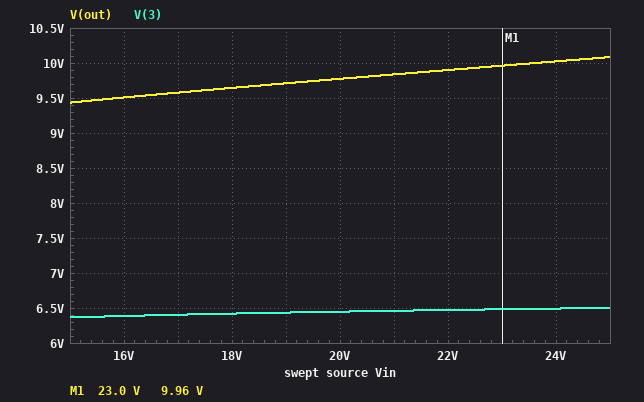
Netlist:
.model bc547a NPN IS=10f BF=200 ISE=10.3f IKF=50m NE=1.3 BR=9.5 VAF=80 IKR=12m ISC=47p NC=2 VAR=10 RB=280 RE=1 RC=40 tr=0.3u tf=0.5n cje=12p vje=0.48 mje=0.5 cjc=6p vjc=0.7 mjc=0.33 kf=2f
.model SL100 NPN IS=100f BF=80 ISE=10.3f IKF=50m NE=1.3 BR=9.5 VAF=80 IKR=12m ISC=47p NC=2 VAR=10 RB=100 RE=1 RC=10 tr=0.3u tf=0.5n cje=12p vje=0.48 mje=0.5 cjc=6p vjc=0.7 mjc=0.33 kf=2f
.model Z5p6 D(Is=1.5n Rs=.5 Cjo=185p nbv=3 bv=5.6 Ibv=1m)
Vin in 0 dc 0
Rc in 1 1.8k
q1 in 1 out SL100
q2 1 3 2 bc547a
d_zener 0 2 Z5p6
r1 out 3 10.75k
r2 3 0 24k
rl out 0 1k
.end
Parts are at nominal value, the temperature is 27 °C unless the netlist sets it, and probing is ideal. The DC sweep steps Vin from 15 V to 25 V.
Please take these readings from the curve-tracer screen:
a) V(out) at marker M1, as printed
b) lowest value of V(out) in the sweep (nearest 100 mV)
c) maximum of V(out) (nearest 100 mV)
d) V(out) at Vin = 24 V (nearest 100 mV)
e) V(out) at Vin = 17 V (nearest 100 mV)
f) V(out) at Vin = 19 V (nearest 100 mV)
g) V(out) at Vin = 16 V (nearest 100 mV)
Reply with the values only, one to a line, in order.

9.96 V
9.4 V
10.1 V
10.0 V
9.6 V
9.7 V
9.5 V
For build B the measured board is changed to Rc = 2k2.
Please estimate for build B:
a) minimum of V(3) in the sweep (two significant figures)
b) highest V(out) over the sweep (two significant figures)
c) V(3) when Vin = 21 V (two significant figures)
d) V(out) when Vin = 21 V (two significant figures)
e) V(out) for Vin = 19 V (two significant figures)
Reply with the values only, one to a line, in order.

6.3 V
9.9 V
6.4 V
9.7 V
9.6 V
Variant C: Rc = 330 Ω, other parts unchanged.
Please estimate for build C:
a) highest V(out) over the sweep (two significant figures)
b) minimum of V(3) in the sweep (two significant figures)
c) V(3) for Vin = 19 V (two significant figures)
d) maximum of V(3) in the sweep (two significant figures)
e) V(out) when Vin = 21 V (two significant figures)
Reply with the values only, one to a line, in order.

13 V
6.6 V
6.7 V
6.8 V
12 V
